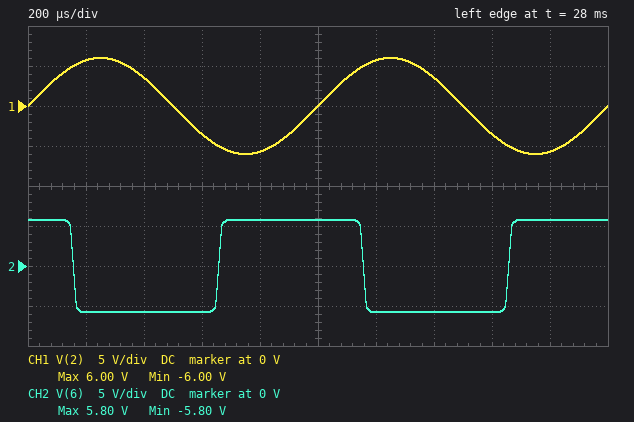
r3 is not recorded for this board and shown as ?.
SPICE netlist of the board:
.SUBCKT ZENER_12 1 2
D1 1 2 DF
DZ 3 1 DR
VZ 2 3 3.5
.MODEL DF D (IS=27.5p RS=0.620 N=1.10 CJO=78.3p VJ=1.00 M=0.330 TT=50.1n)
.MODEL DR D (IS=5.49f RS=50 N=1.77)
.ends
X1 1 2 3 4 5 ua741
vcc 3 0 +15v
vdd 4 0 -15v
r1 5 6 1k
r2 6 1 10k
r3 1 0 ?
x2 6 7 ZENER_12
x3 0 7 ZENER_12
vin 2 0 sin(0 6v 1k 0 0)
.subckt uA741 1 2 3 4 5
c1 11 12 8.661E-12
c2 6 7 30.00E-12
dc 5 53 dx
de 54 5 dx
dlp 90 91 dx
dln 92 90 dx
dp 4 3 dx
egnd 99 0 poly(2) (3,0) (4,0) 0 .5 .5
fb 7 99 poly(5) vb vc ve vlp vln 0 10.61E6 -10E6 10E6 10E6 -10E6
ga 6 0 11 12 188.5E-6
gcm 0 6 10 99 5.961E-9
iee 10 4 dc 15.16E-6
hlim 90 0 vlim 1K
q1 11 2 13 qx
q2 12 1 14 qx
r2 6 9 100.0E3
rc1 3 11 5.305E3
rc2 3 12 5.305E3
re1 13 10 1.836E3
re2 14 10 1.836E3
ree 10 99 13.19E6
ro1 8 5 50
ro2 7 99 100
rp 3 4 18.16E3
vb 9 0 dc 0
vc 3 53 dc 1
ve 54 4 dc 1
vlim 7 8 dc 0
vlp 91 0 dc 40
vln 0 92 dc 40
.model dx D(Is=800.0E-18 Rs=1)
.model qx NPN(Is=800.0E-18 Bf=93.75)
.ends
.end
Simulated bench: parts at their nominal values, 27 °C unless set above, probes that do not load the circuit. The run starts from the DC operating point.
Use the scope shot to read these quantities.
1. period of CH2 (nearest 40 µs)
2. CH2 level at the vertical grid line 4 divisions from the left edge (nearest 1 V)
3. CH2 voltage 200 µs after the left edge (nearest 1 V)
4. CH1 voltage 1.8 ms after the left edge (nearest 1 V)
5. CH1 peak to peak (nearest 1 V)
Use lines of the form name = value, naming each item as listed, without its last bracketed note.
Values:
period of CH2 = 1.00 ms
CH2 level at the vertical grid line 4 divisions from the left edge = 6 V
CH2 voltage 200 µs after the left edge = -6 V
CH1 voltage 1.8 ms after the left edge = -6 V
CH1 peak to peak = 12 V
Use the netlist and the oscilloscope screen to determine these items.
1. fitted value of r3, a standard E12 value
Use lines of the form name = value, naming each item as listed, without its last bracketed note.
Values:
fitted value of r3, a standard E12 value = 27 kΩ
